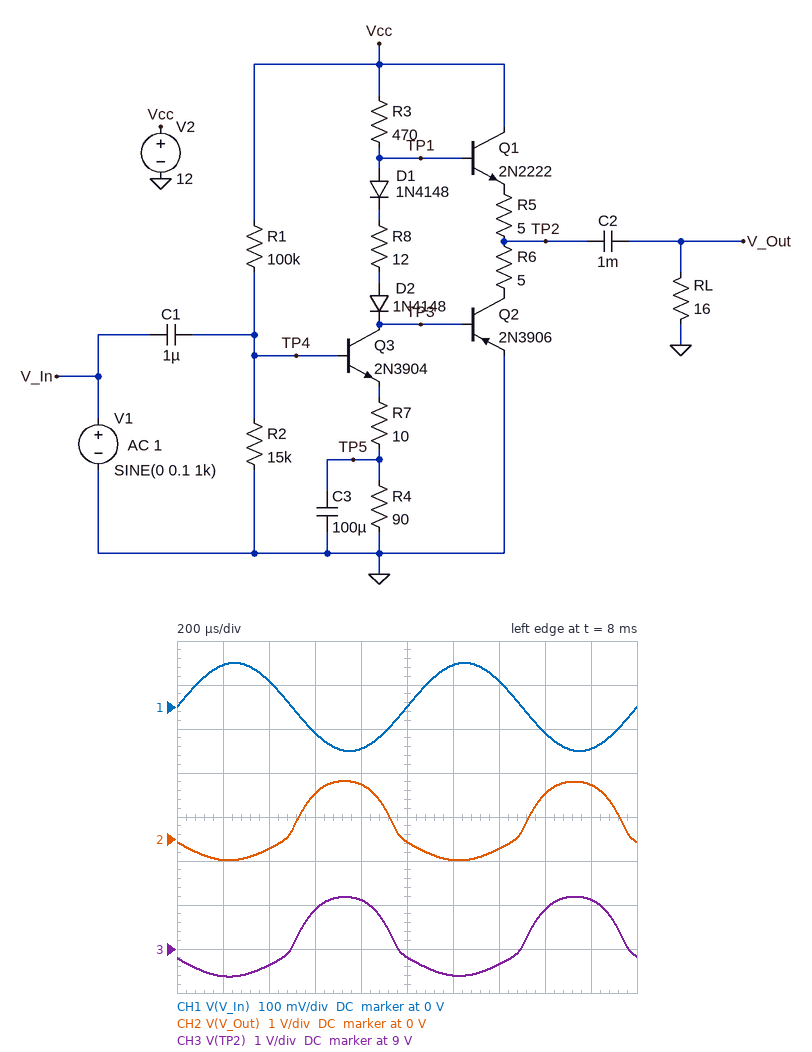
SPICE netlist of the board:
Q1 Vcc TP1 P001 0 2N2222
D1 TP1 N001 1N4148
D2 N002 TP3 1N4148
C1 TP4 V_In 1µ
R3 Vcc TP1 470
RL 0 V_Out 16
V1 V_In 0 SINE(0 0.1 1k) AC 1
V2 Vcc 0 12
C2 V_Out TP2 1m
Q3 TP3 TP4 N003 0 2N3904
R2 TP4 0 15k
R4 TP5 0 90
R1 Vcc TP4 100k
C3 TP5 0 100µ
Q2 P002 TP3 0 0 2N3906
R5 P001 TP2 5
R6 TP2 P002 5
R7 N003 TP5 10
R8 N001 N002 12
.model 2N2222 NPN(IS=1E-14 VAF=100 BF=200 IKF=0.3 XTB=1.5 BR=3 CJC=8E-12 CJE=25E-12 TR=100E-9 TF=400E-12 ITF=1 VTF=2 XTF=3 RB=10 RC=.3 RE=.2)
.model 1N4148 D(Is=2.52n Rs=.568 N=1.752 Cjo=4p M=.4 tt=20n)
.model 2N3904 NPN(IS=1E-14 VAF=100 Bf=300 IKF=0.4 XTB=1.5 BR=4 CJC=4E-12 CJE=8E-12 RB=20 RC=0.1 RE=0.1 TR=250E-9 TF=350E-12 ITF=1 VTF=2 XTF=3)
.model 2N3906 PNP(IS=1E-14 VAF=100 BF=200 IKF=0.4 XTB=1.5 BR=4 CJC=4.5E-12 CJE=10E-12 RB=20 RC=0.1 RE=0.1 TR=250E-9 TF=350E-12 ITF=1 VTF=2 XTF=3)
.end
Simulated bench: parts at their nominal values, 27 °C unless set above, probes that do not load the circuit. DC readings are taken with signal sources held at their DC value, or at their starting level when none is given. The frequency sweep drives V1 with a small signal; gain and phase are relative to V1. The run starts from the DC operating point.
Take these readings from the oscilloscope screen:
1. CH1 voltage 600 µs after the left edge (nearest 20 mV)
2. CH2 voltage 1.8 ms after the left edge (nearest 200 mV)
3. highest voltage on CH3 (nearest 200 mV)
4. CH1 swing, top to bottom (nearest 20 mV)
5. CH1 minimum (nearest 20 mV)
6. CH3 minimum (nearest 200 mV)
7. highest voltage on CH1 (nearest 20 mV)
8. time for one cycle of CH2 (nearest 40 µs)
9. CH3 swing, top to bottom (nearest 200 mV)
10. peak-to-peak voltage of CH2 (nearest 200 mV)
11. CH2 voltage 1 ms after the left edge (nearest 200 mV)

-60 mV
1.2 V
10.2 V
200 mV
-100 mV
8.4 V
100 mV
1.00 ms
1.8 V
1.8 V
0 V
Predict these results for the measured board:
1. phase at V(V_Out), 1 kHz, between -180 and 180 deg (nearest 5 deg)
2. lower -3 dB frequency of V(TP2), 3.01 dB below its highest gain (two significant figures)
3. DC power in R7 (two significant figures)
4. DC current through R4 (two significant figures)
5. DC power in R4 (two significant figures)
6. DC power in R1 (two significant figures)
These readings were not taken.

-170 deg
160 Hz
370 µW
6.1 mA
3.4 mW
1.1 mW
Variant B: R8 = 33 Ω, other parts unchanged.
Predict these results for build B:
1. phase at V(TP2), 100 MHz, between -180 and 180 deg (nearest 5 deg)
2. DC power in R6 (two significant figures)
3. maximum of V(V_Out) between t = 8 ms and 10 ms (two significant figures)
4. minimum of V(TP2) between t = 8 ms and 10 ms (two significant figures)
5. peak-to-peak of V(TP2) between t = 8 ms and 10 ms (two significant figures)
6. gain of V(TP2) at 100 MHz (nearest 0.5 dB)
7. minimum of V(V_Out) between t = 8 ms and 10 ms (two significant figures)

110 deg
170 µW
1.2 V
8.5 V
1.7 V
1.0 dB
-530 mV
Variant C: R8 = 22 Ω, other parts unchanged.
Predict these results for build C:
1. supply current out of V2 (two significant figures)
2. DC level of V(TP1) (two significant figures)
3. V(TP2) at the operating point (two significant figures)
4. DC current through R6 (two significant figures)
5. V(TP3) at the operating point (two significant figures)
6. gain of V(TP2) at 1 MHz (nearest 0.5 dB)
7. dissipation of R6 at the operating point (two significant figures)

9.6 mA
9.5 V
8.8 V
4.2 mA
8.1 V
9.5 dB
90 µW
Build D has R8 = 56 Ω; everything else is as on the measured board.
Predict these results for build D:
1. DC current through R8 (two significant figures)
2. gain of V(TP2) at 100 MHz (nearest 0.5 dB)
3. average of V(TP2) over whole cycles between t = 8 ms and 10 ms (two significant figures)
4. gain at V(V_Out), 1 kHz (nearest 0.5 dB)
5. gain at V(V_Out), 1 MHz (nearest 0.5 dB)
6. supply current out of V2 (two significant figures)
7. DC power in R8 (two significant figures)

4.3 mA
0.5 dB
9.4 V
16.5 dB
9.5 dB
13 mA
1.0 mW
